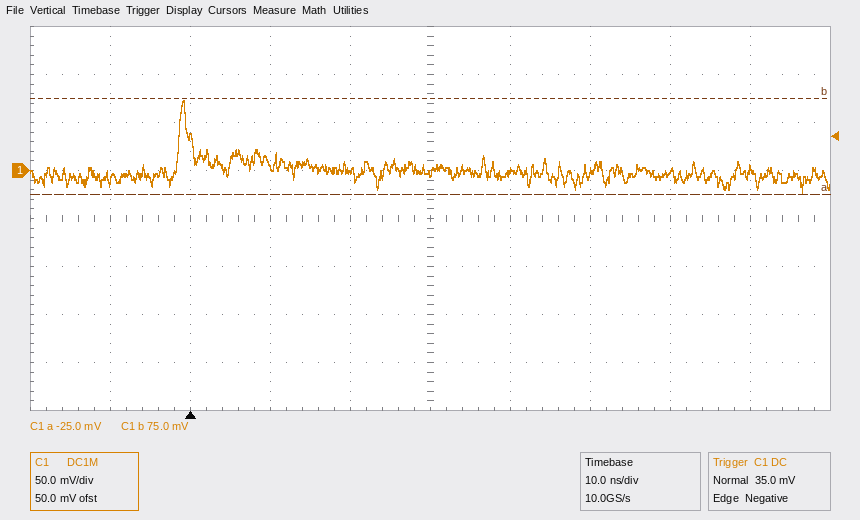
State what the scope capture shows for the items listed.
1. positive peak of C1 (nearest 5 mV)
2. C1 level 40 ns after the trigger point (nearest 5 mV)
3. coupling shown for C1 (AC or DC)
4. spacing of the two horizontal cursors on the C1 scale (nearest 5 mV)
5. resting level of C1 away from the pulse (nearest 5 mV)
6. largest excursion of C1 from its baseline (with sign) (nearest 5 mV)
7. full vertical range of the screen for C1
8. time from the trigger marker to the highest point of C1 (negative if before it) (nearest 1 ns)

75 mV
0 mV
DC
100 mV
0 mV
+75 mV
400 mV
-1 ns
